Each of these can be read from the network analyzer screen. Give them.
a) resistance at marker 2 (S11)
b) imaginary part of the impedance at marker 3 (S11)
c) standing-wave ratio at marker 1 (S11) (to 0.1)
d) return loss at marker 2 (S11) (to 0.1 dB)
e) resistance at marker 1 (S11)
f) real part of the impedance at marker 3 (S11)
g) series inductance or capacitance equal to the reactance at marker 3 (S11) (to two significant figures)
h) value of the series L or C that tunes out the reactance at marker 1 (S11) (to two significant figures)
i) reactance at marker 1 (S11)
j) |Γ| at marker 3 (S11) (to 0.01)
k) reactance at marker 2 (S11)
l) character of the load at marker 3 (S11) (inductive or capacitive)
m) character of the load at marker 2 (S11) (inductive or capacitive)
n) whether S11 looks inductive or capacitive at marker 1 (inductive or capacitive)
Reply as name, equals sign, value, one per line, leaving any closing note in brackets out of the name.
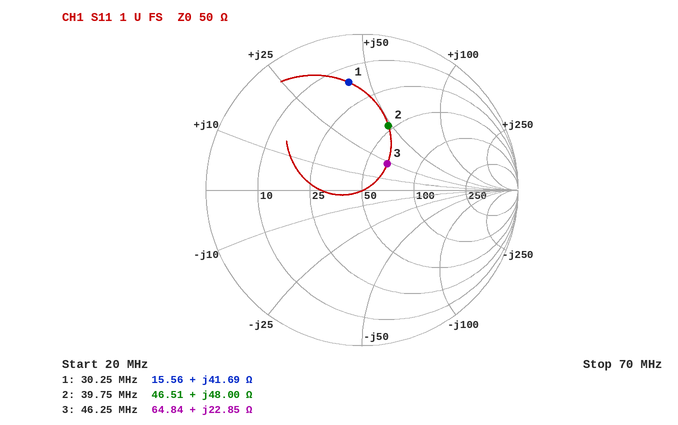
resistance at marker 2 = 46.51 Ω
imaginary part of the impedance at marker 3 = +22.85 Ω
standing-wave ratio at marker 1 (S11) = 5.6
return loss at marker 2 (S11) = 7.0 dB
resistance at marker 1 = 15.56 Ω
real part of the impedance at marker 3 = 64.84 Ω
series inductance or capacitance equal to the reactance at marker 3 (S11) = 79 nH
value of the series L or C that tunes out the reactance at marker 1 (S11) = 130 pF
reactance at marker 1 = +41.69 Ω
|Γ| at marker 3 (S11) = 0.23
reactance at marker 2 = +48.00 Ω
character of the load at marker 3 (S11) = inductive
character of the load at marker 2 (S11) = inductive
whether S11 looks inductive or capacitive at marker 1 = inductive
